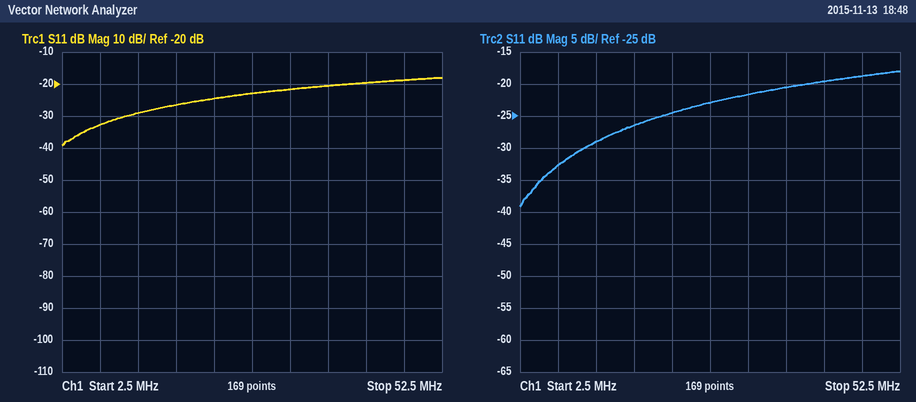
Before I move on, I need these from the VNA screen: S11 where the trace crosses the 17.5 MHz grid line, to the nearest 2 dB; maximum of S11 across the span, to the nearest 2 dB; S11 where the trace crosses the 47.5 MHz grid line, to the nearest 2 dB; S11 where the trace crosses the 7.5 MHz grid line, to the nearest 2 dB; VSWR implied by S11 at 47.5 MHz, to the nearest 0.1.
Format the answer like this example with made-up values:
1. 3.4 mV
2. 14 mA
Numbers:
1. -26 dB
2. -18 dB
3. -18 dB
4. -32 dB
5. 1.3
